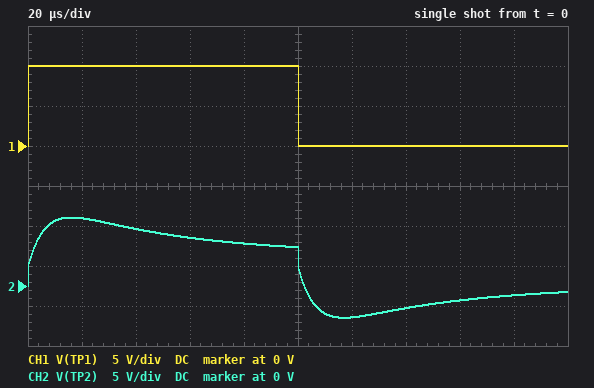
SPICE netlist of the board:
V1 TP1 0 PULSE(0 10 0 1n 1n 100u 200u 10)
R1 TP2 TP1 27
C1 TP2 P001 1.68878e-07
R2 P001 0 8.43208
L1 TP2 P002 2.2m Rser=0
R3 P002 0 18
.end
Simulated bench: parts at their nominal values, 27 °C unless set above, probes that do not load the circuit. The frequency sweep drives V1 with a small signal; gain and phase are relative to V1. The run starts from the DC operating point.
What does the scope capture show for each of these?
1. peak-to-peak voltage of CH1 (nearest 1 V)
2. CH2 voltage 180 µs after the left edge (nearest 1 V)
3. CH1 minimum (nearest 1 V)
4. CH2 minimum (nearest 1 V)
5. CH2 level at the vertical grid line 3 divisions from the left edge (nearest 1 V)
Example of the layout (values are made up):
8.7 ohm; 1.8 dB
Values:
10 V; -1 V; 0 V; -4 V; 6 V
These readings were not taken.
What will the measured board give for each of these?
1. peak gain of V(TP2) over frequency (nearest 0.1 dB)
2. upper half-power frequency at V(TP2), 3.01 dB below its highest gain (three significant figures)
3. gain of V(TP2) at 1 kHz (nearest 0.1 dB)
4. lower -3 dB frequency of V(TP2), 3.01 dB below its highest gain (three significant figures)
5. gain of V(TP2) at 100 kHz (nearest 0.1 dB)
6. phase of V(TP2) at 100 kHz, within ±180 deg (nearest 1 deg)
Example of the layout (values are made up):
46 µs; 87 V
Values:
-0.4 dB; 32.6 kHz; -6.3 dB; 2.28 kHz; -9.2 dB; -33 deg
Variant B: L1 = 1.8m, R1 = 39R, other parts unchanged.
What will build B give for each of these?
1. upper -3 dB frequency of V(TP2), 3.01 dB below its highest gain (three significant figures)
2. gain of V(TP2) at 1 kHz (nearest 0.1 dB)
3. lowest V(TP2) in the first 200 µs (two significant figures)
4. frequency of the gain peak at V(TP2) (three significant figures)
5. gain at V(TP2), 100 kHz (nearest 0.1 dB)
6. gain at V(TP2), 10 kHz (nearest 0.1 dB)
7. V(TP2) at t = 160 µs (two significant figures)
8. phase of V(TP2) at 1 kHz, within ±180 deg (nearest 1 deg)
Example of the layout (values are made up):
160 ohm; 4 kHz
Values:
26.4 kHz; -8.7 dB; -4.4 V; 9.79 kHz; -11.6 dB; -0.8 dB; -1.3 V; 20 deg
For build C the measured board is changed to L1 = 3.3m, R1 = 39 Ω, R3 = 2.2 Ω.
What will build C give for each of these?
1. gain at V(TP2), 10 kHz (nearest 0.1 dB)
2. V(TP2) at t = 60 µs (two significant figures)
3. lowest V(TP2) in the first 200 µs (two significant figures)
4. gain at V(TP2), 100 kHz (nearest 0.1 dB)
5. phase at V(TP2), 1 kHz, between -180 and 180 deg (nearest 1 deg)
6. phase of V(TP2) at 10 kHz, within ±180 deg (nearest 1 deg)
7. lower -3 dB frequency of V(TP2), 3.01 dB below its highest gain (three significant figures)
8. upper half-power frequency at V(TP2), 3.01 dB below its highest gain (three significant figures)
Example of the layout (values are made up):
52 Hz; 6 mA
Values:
-0.5 dB; 5.6 V; -5.6 V; -11.6 dB; 57 deg; -12 deg; 1.79 kHz; 22.8 kHz
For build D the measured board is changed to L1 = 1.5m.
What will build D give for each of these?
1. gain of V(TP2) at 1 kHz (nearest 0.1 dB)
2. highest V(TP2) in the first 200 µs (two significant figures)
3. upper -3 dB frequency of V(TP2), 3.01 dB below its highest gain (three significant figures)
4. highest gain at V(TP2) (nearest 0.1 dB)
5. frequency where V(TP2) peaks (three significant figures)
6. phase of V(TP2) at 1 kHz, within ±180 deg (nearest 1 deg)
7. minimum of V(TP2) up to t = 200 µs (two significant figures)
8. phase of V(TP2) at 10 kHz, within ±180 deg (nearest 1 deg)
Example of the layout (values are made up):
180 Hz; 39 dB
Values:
-7.1 dB; 8.2 V; 34.5 kHz; -0.6 dB; 10.9 kHz; 15 deg; -4.0 V; 0 deg
